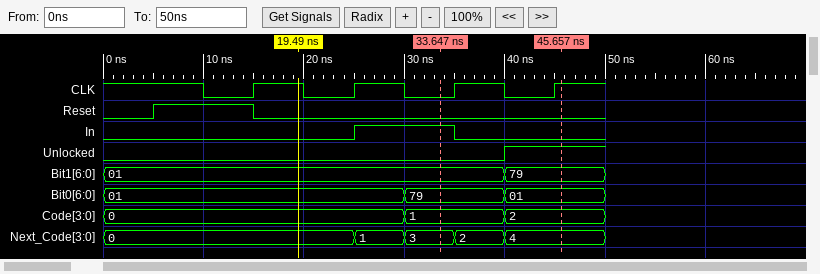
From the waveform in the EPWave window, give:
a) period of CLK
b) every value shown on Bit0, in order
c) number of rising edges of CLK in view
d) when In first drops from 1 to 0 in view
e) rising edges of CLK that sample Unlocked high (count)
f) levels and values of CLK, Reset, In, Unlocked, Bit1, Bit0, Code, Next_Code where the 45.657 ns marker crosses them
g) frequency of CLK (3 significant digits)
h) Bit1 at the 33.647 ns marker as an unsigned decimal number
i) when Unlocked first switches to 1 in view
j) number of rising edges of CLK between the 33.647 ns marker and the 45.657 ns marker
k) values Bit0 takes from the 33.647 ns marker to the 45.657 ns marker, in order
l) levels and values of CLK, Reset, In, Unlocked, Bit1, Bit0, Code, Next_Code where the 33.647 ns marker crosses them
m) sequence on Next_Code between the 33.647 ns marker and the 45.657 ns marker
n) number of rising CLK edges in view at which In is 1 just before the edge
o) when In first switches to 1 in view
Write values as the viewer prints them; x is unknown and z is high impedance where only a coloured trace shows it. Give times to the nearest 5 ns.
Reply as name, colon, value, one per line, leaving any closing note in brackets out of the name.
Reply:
period of CLK: 10 ns
every value shown on Bit0, in order: 01, 79, 01
number of rising edges of CLK in view: 4
when In first drops from 1 to 0 in view: 35 ns
rising edges of CLK that sample Unlocked high: 1
levels and values of CLK, Reset, In, Unlocked, Bit1, Bit0, Code, Next_Code where the 45.657 ns marker crosses them: CLK=1, Reset=0, In=0, Unlocked=1, Bit1=79, Bit0=01, Code=2, Next_Code=4
frequency of CLK: 100 MHz
Bit1 at the 33.647 ns marker as an unsigned decimal number: 1
when Unlocked first switches to 1 in view: 40 ns
number of rising edges of CLK between the 33.647 ns marker and the 45.657 ns marker: 2
values Bit0 takes from the 33.647 ns marker to the 45.657 ns marker, in order: 79, 01
levels and values of CLK, Reset, In, Unlocked, Bit1, Bit0, Code, Next_Code where the 33.647 ns marker crosses them: CLK=0, Reset=0, In=1, Unlocked=0, Bit1=01, Bit0=79, Code=1, Next_Code=3
sequence on Next_Code between the 33.647 ns marker and the 45.657 ns marker: 3, 2, 4
number of rising CLK edges in view at which In is 1 just before the edge: 1
when In first switches to 1 in view: 25 ns
